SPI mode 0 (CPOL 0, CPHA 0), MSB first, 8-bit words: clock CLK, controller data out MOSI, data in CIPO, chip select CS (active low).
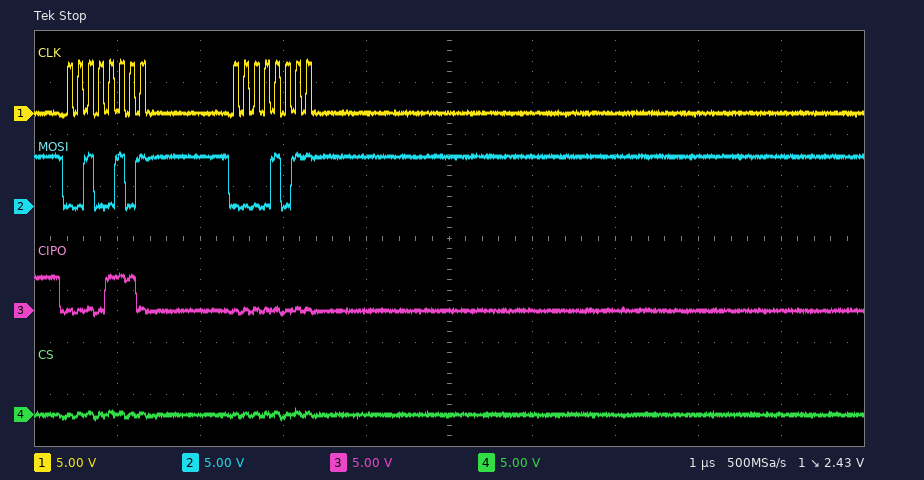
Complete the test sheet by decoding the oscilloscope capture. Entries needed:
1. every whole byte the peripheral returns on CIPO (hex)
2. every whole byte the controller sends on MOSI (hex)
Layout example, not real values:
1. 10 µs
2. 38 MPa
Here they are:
1. 0E 00
2. 25 0B
